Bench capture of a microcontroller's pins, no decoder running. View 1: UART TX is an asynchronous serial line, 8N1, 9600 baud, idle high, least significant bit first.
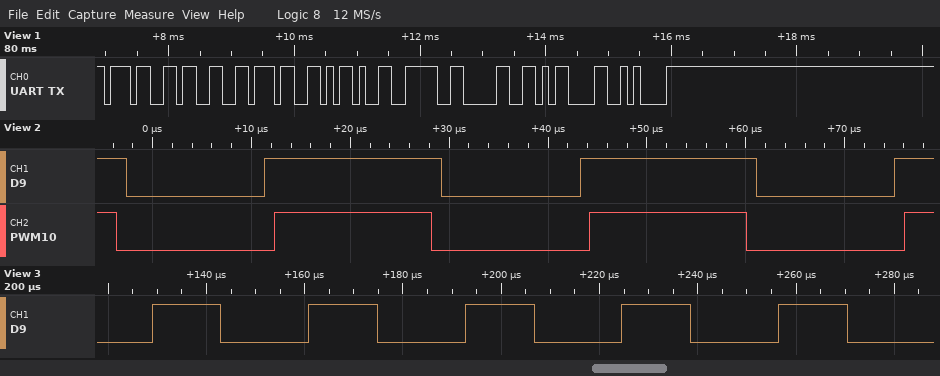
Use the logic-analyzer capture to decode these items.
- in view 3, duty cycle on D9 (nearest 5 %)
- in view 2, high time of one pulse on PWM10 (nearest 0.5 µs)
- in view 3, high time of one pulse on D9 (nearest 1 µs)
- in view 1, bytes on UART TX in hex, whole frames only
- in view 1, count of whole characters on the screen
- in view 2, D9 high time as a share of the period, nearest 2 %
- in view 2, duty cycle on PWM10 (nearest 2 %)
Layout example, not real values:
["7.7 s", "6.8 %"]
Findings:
["45 %", "16.0 µs", "14 µs", "37 33 37 2D 3E 30 0D 0A", "8", "56 %", "50 %"]
